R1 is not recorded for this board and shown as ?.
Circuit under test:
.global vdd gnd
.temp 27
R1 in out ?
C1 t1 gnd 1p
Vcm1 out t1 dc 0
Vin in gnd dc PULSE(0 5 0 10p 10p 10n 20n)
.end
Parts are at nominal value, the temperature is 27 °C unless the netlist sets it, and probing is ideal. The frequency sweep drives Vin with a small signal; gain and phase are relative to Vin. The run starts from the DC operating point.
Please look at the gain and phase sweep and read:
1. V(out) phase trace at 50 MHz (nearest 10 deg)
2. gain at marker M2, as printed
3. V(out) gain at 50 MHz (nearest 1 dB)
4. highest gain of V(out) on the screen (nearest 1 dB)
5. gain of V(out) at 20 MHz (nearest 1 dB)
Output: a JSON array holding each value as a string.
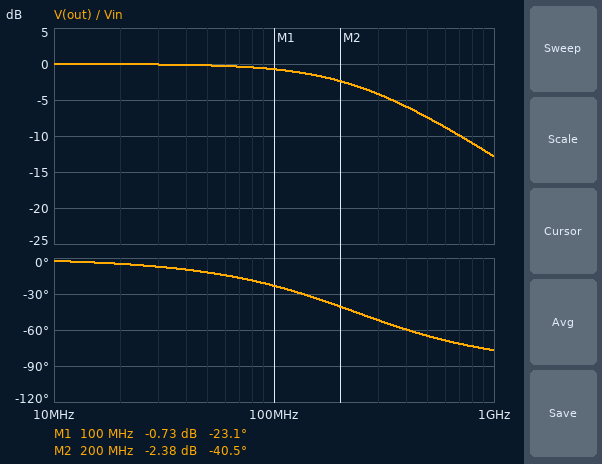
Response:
["-10 deg", "-2.38 dB", "0 dB", "0 dB", "0 dB"]
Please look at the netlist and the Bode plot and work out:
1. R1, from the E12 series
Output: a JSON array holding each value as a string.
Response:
["680 Ω"]
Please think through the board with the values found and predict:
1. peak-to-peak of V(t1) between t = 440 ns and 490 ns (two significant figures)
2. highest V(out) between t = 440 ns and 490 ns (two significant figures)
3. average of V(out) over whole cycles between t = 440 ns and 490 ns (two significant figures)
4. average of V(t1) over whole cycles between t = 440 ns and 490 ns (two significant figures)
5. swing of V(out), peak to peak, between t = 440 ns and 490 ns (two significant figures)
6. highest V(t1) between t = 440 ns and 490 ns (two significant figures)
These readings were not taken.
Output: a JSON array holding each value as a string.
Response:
["5.0 V", "5.0 V", "2.5 V", "2.5 V", "5.0 V", "5.0 V"]
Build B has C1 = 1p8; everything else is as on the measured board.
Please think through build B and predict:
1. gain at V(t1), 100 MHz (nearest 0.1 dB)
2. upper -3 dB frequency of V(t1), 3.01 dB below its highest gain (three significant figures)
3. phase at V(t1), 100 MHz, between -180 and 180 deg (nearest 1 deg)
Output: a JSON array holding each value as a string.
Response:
["-2.0 dB", "130 MHz", "-38 deg"]
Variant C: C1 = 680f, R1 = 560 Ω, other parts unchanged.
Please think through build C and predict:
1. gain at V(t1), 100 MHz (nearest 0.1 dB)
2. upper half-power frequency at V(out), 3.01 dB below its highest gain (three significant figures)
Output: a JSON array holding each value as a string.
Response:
["-0.2 dB", "418 MHz"]
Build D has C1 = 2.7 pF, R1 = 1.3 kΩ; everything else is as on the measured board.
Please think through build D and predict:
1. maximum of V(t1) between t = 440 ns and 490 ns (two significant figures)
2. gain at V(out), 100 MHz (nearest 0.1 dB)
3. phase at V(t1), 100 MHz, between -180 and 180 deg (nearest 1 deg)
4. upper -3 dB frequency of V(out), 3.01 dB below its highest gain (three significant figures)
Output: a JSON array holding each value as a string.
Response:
["4.7 V", "-7.7 dB", "-66 deg", "45.3 MHz"]
